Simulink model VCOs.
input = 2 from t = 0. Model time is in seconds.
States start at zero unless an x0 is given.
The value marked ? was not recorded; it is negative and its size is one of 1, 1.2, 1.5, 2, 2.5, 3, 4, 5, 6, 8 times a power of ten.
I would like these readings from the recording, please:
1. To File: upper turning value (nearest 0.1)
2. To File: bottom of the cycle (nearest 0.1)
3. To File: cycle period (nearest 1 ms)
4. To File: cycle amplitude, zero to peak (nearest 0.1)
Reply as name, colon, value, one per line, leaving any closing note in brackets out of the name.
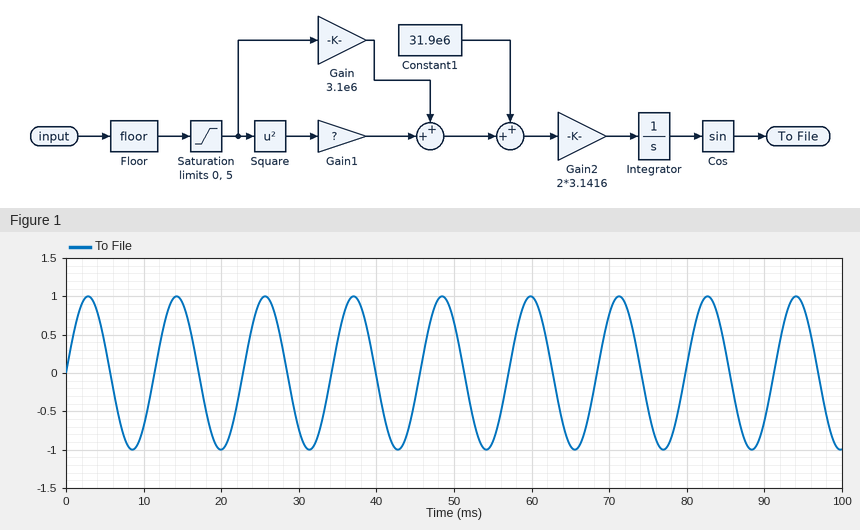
To File: upper turning value: 1.0
To File: bottom of the cycle: -1.0
To File: cycle period: 11 ms
To File: cycle amplitude, zero to peak: 1.0
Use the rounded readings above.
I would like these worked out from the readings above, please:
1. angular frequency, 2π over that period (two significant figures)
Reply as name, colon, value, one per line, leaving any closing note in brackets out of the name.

angular frequency, 2π over that period: 0.57 rad/ms
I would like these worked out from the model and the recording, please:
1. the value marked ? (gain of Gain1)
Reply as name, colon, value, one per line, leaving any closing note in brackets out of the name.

the value marked ?: -150000
